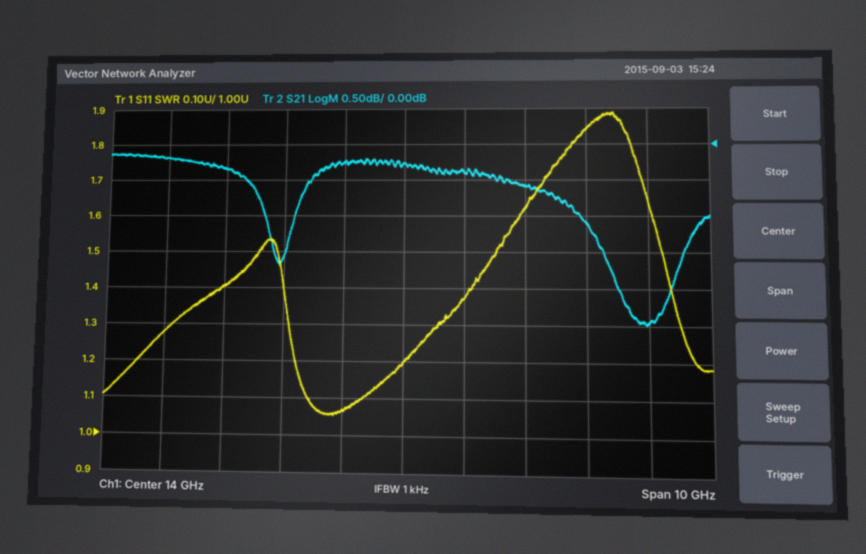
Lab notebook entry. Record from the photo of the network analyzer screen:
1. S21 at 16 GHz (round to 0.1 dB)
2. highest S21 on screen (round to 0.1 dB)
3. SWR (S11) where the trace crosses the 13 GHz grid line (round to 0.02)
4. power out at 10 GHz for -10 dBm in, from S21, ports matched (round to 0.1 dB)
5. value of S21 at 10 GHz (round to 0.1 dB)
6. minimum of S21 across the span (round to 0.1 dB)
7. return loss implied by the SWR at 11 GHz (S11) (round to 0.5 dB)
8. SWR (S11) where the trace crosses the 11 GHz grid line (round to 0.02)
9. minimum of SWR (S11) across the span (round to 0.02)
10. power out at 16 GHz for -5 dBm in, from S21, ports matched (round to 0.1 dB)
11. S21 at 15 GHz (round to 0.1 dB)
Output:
-0.6 dB
-0.1 dB
1.06
-10.2 dBm
-0.2 dB
-2.5 dB
15.5 dB
1.40
1.06
-5.6 dBm
-0.4 dB
